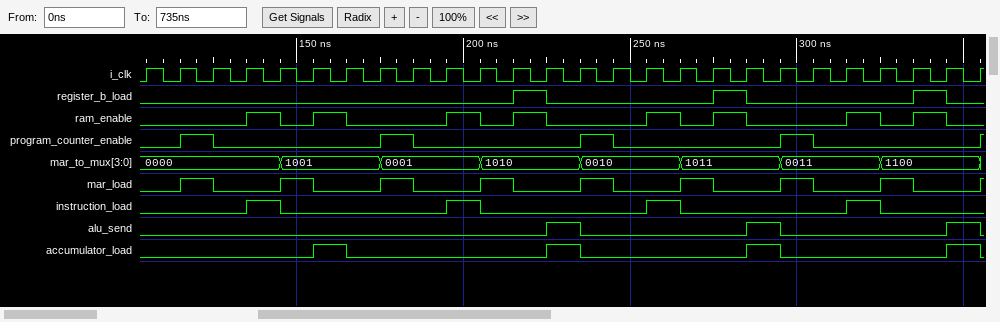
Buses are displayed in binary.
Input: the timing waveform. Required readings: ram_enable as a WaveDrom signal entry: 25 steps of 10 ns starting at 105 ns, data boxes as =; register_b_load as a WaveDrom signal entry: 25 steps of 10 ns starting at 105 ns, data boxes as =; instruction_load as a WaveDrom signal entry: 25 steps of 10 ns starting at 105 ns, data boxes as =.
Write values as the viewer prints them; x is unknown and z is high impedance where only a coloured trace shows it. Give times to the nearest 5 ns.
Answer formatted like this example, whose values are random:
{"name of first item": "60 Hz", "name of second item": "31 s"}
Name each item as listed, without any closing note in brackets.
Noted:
{"ram_enable as a WaveDrom signal entry: 25 steps of 10 ns starting at 105 ns, data boxes as =": "{name: 'ram_enable', wave: '0..1010..1010..1010..1010'}", "register_b_load as a WaveDrom signal entry: 25 steps of 10 ns starting at 105 ns, data boxes as =": "{name: 'register_b_load', wave: '0..........10....10....10'}", "instruction_load as a WaveDrom signal entry: 25 steps of 10 ns starting at 105 ns, data boxes as =": "{name: 'instruction_load', wave: '0..10....10....10....10..'}"}
